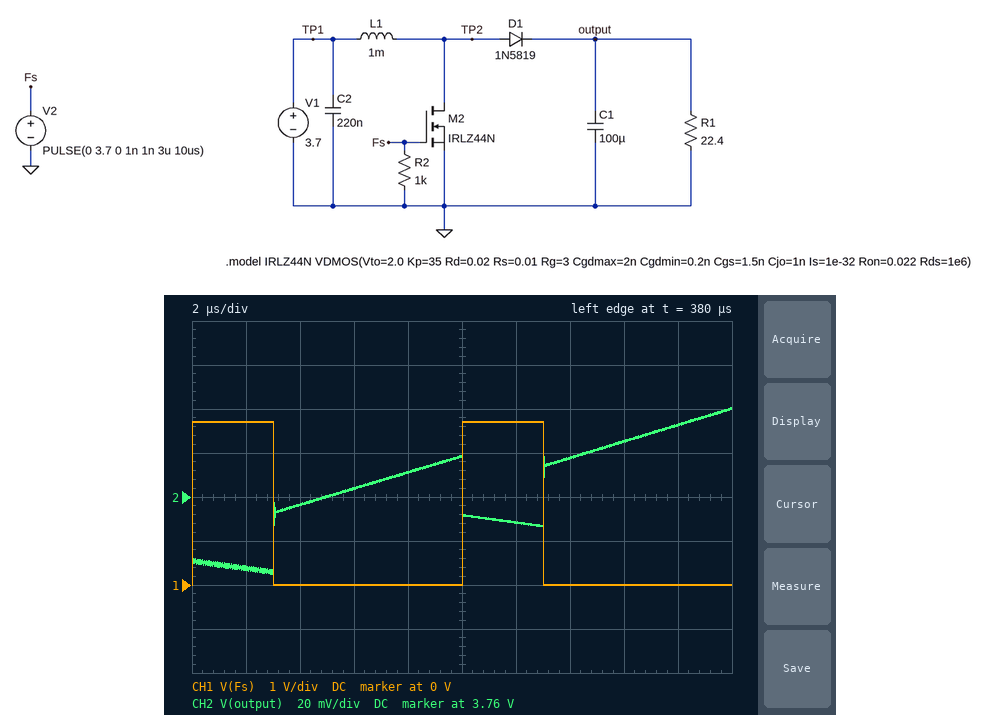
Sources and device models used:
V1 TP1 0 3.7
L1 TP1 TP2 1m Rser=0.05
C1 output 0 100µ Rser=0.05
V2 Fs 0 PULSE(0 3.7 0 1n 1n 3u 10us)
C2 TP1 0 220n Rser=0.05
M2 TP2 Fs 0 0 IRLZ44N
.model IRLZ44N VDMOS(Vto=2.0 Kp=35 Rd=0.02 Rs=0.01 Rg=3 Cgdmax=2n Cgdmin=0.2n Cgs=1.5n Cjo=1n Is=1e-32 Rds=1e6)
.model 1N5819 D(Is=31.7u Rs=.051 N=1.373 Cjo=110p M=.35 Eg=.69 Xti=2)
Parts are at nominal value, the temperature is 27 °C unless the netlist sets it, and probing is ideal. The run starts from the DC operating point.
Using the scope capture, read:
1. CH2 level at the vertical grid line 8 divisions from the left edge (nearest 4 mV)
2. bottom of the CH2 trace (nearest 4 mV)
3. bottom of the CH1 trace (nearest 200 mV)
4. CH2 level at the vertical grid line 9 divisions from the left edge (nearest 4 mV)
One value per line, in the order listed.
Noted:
3.784 V
3.724 V
0 V
3.792 V
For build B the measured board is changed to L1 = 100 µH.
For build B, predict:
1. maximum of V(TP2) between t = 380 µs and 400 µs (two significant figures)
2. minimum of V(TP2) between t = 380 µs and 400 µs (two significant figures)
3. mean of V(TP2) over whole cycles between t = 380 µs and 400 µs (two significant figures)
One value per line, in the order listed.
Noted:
6.2 V
18 mV
4.3 V
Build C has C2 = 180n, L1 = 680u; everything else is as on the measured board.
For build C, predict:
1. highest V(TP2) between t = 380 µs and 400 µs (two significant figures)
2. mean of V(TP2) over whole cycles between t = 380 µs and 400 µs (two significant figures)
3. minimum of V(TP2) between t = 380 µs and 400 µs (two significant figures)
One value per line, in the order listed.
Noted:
4.5 V
3.1 V
9.4 mV
